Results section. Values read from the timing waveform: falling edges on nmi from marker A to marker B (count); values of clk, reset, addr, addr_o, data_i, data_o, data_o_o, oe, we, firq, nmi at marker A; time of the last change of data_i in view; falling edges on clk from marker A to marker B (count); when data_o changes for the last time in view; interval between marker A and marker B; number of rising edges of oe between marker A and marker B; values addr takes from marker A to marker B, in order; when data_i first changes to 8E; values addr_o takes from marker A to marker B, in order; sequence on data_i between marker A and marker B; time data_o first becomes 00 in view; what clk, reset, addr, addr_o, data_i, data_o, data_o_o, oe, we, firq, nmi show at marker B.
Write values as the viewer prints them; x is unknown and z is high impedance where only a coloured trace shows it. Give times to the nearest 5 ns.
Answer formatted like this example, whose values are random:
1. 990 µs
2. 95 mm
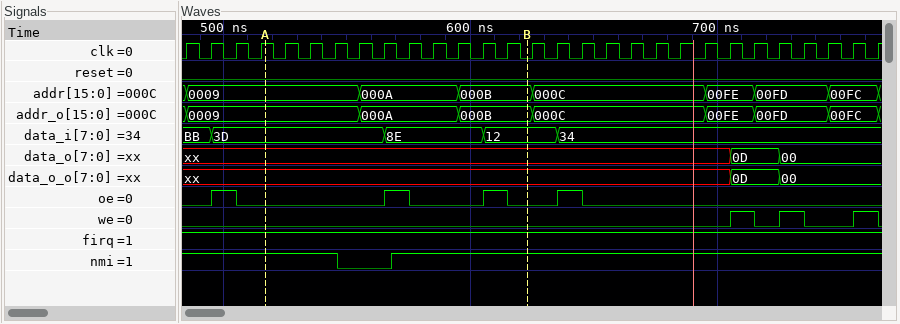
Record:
1. 1
2. clk=1, reset=0, addr=0009, addr_o=0009, data_i=3D, data_o=xx, data_o_o=xx, oe=0, we=0, firq=1, nmi=1
3. 635 ns
4. 11
5. 725 ns
6. 105 ns
7. 2
8. 0009, 000A, 000B
9. 565 ns
10. 0009, 000A, 000B
11. 3D, 8E, 12
12. 725 ns
13. clk=0, reset=0, addr=000B, addr_o=000B, data_i=12, data_o=xx, data_o_o=xx, oe=0, we=0, firq=1, nmi=1
